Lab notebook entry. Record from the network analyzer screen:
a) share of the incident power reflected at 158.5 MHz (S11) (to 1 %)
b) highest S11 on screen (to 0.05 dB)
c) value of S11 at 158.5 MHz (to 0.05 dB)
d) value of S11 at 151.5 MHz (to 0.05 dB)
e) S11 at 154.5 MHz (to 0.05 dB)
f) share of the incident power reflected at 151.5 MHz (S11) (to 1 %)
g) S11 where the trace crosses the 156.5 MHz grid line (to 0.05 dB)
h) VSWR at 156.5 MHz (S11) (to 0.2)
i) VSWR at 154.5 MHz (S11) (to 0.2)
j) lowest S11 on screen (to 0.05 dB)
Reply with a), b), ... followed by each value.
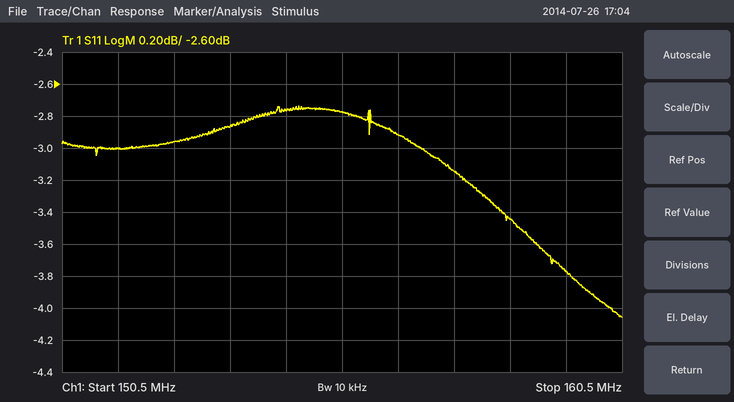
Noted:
a) 45 %
b) -2.75 dB
c) -3.45 dB
d) -3.00 dB
e) -2.75 dB
f) 50 %
g) -2.90 dB
h) 6.0
i) 6.4
j) -4.05 dB
